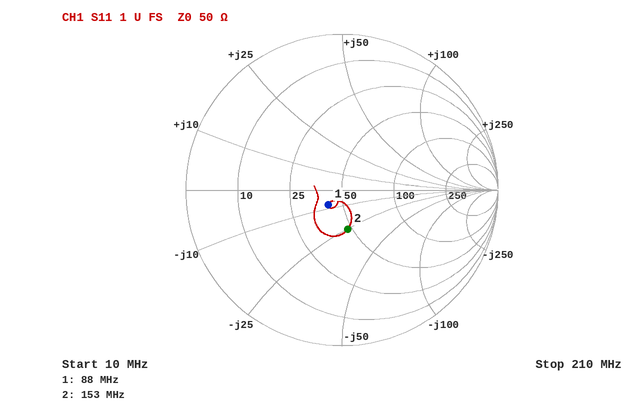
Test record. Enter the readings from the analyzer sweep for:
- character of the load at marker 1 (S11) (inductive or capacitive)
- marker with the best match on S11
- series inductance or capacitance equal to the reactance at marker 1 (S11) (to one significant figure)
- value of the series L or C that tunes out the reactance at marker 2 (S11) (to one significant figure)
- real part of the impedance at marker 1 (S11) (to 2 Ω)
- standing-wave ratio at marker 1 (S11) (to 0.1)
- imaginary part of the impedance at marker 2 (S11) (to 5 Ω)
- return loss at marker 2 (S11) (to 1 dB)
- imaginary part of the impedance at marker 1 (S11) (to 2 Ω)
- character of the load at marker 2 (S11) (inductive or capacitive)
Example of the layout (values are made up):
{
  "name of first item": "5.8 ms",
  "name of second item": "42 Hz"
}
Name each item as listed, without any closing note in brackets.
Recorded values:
{
  "character of the load at marker 1 (S11)": "capacitive",
  "marker with the best match on S11": "marker 1",
  "series inductance or capacitance equal to the reactance at marker 1 (S11)": "200 pF",
  "value of the series L or C that tunes out the reactance at marker 2 (S11)": "30 nH",
  "real part of the impedance at marker 1 (S11)": "42 Ω",
  "standing-wave ratio at marker 1 (S11)": "1.3",
  "imaginary part of the impedance at marker 2 (S11)": "-25 Ω",
  "return loss at marker 2 (S11)": "12 dB",
  "imaginary part of the impedance at marker 1 (S11)": "-8 Ω",
  "character of the load at marker 2 (S11)": "capacitive"
}
